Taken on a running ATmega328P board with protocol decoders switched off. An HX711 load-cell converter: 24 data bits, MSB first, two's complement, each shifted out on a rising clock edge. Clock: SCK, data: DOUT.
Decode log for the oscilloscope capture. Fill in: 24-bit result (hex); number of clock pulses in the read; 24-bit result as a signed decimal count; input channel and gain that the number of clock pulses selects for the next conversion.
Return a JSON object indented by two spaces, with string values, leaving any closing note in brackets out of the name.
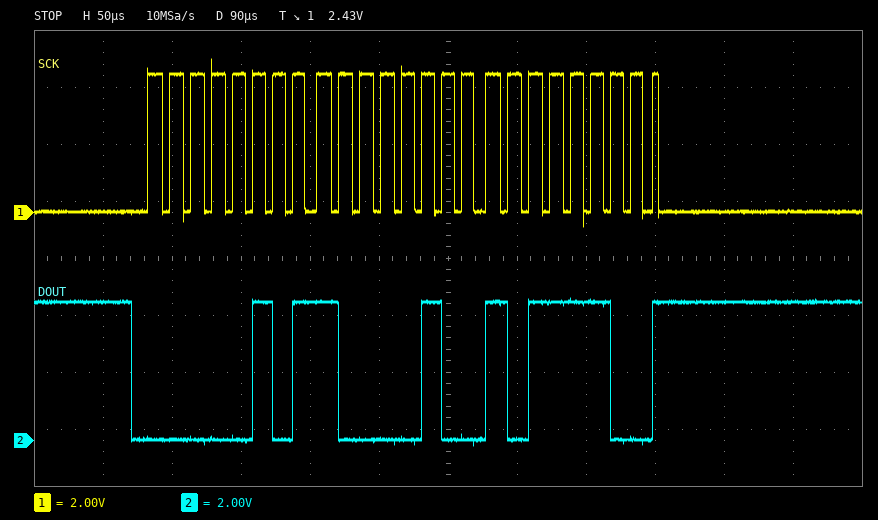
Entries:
{
  "24-bit result": "0x0584BC",
  "number of clock pulses in the read": "25",
  "24-bit result as a signed decimal count": "361660",
  "input channel and gain that the number of clock pulses selects for the next conversion": "channel A, gain 128"
}
